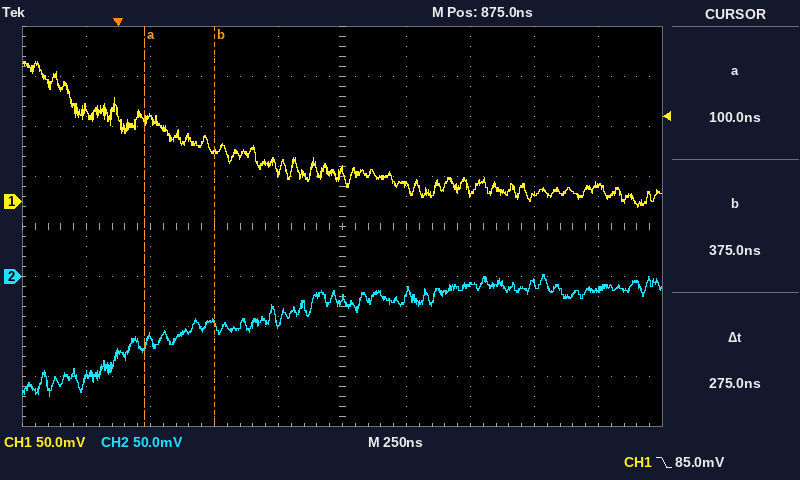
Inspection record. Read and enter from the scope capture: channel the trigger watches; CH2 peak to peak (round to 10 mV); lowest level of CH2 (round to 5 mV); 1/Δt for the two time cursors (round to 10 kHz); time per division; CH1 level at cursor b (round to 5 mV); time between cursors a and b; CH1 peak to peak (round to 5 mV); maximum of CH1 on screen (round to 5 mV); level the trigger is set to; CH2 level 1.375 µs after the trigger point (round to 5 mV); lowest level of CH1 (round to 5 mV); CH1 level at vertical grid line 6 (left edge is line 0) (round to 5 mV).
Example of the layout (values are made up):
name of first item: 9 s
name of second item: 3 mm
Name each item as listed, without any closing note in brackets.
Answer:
channel the trigger watches: CH1
CH2 peak to peak: 120 mV
lowest level of CH2: -120 mV
1/Δt for the two time cursors: 3.64 MHz
time per division: 250 ns
CH1 level at cursor b: 50 mV
time between cursors a and b: 275 ns
CH1 peak to peak: 145 mV
maximum of CH1 on screen: 140 mV
level the trigger is set to: 85.0 mV
CH2 level 1.375 µs after the trigger point: -10 mV
lowest level of CH1: -5 mV
CH1 level at vertical grid line 6 (left edge is line 0): 15 mV
